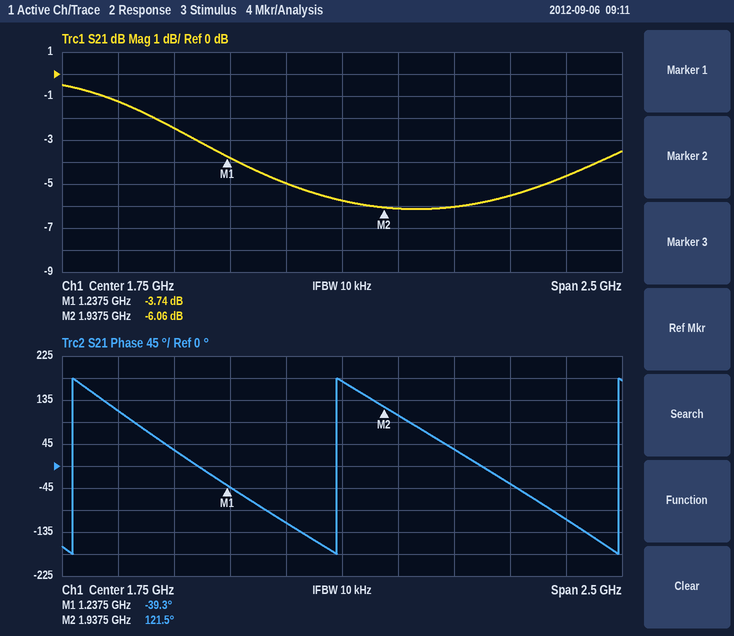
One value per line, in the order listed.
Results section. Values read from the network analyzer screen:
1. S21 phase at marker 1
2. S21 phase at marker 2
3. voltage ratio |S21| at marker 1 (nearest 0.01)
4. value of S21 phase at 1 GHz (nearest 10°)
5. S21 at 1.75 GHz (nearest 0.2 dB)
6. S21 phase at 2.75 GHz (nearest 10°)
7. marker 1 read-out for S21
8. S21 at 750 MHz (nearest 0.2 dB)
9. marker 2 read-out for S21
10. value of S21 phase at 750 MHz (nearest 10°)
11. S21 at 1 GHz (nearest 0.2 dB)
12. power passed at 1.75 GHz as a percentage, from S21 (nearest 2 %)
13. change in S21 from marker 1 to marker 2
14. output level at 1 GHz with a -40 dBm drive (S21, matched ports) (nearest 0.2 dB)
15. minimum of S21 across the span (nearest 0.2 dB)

-39.3°
121.5°
0.65
30°
-5.8 dB
-110°
-3.74 dB
-1.2 dB
-6.06 dB
110°
-2.4 dB
26 %
-2.32 dB
-42.4 dBm
-6.2 dB
